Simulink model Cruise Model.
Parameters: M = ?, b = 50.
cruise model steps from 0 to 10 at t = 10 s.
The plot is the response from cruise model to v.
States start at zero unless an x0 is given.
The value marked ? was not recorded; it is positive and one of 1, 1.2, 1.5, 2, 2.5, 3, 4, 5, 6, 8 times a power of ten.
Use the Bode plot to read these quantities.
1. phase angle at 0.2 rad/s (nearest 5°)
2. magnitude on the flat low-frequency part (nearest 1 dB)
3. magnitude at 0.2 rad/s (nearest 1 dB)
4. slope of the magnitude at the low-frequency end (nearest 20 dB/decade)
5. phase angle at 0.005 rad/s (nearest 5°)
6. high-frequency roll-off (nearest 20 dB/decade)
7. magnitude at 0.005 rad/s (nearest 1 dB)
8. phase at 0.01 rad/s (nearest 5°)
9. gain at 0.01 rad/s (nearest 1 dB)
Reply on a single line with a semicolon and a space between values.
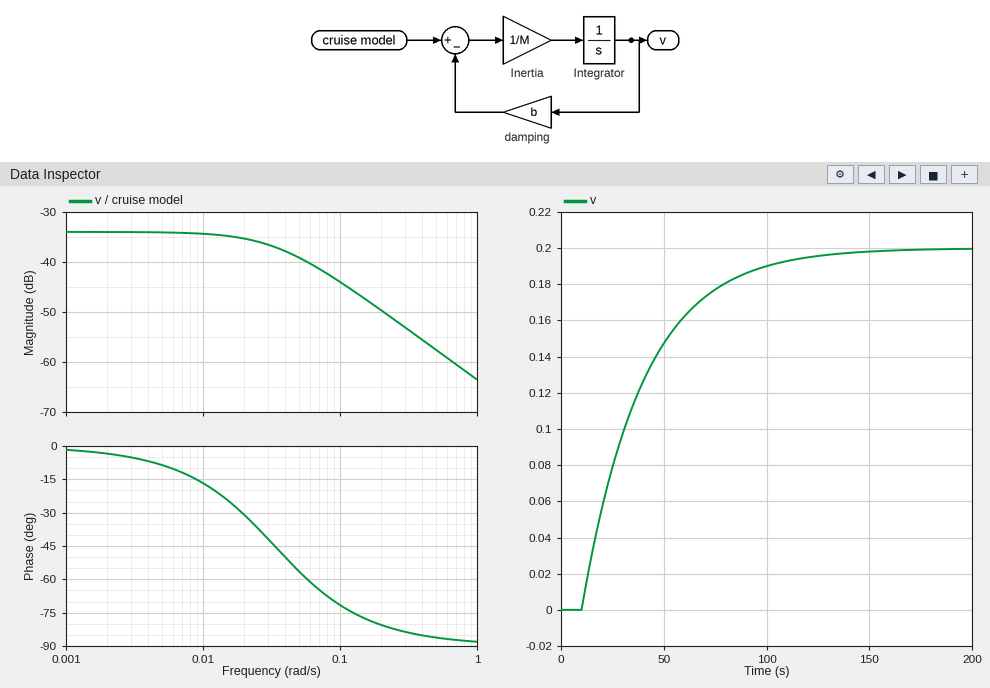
-80°; -34 dB; -50 dB; 0 dB/decade; -10°; -20 dB/decade; -34 dB; -15°; -34 dB
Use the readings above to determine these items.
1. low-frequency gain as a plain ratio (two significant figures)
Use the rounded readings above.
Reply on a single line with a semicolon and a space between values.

0.020
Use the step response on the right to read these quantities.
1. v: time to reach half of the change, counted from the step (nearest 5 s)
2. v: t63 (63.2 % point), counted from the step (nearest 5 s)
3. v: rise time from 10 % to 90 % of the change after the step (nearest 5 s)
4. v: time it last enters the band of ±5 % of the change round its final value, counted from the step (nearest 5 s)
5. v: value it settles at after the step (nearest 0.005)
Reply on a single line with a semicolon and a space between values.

20 s; 30 s; 65 s; 90 s; 0.200
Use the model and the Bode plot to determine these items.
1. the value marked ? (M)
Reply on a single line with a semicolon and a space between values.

1500
